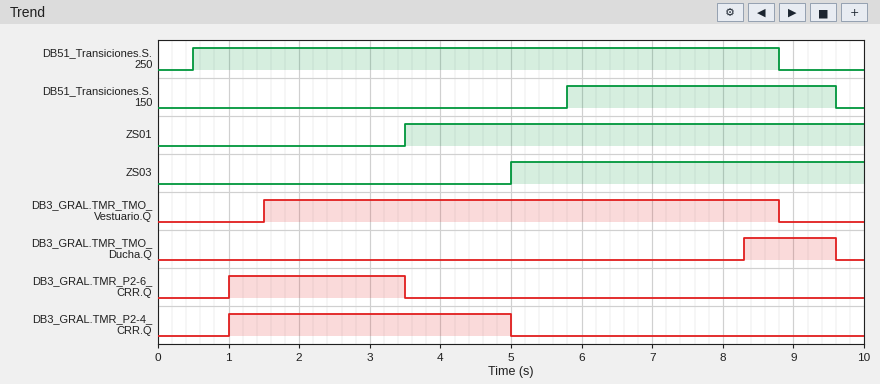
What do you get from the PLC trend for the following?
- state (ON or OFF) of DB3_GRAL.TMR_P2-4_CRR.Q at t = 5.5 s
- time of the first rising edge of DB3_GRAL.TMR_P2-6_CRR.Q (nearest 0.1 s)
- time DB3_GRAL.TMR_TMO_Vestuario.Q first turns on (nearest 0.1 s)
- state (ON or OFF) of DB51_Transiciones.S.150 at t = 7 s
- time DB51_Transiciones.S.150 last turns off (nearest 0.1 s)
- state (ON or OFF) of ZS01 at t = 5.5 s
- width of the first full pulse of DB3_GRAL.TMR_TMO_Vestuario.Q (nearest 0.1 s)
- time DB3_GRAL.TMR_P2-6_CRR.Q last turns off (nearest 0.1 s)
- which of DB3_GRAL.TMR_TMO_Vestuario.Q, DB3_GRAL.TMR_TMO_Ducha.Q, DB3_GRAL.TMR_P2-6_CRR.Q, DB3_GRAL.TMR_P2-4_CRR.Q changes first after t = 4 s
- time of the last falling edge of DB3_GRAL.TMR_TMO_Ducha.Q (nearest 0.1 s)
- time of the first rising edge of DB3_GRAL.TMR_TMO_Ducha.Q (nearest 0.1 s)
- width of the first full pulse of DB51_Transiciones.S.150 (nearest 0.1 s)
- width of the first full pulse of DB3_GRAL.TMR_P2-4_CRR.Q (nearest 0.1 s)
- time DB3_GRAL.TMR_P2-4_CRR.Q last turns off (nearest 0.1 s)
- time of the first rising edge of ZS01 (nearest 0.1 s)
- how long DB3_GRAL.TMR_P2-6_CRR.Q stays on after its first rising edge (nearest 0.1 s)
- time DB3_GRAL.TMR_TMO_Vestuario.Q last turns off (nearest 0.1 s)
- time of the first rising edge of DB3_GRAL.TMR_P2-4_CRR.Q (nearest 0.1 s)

OFF
1.0 s
1.5 s
ON
9.6 s
ON
7.3 s
3.5 s
DB3_GRAL.TMR_P2-4_CRR.Q
9.6 s
8.3 s
3.8 s
4.0 s
5.0 s
3.5 s
2.5 s
8.8 s
1.0 s
